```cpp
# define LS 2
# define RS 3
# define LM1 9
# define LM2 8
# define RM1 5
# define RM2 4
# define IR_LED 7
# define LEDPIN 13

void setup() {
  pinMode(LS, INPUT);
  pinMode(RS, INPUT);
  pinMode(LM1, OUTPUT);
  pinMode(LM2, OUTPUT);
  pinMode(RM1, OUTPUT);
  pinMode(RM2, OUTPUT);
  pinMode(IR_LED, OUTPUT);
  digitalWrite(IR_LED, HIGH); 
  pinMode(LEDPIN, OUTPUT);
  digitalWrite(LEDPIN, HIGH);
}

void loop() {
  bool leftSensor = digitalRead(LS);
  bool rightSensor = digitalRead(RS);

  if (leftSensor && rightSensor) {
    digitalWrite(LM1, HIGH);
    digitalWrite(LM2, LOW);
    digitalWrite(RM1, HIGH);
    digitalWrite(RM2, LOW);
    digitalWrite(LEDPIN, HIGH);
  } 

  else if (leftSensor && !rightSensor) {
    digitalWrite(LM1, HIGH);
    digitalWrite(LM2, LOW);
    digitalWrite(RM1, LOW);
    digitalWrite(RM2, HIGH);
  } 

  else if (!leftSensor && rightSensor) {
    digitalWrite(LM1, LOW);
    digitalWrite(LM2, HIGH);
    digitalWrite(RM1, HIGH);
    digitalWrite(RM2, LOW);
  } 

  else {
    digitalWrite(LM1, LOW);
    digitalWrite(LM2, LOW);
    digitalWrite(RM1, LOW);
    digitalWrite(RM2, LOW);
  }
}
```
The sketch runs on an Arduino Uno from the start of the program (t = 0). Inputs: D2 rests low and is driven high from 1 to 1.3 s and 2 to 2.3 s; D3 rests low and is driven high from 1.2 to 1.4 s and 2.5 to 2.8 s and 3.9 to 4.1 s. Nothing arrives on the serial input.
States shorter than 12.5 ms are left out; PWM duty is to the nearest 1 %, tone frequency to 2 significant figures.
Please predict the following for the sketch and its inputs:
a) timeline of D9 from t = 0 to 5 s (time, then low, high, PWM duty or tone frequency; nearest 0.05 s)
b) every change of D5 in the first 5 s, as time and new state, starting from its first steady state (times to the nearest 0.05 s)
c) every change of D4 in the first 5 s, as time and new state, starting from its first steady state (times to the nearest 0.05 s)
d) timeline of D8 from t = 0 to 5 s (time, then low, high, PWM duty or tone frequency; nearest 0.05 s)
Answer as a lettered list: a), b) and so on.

a) 0 s low; 1 s high; 1.3 s low; 2 s high; 2.3 s low
b) 0 s low; 1.2 s high; 1.4 s low; 2.5 s high; 2.8 s low; 3.9 s high; 4.1 s low
c) 0 s low; 1 s high; 1.2 s low; 2 s high; 2.3 s low
d) 0 s low; 1.3 s high; 1.4 s low; 2.5 s high; 2.8 s low; 3.9 s high; 4.1 s low
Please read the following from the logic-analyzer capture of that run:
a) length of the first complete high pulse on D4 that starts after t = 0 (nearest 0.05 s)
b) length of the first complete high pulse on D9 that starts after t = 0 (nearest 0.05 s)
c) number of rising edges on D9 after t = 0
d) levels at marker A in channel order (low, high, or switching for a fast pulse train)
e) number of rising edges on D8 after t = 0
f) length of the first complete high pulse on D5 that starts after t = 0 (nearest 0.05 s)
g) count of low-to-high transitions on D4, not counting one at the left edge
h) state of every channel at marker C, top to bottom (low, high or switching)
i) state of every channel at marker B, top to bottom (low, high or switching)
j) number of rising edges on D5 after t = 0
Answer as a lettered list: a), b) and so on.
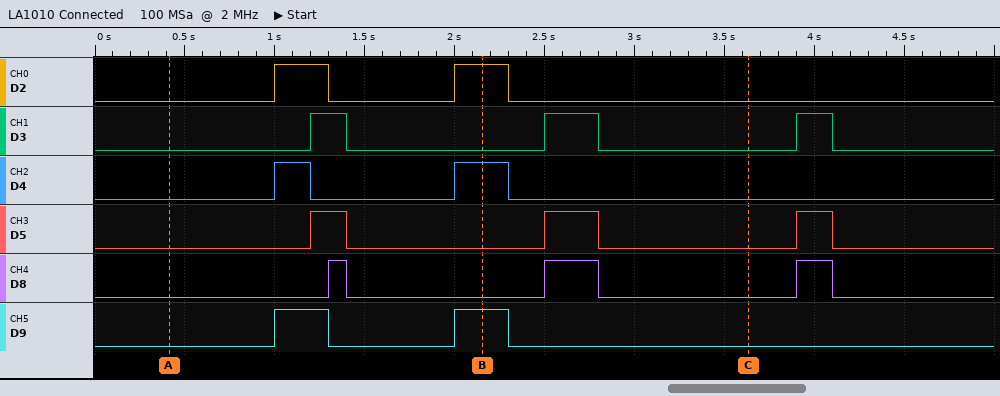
a) 0.20 s
b) 0.30 s
c) 2
d) D2 low, D3 low, D4 low, D5 low, D8 low, D9 low
e) 3
f) 0.20 s
g) 2
h) D2 low, D3 low, D4 low, D5 low, D8 low, D9 low
i) D2 high, D3 low, D4 high, D5 low, D8 low, D9 high
j) 3
